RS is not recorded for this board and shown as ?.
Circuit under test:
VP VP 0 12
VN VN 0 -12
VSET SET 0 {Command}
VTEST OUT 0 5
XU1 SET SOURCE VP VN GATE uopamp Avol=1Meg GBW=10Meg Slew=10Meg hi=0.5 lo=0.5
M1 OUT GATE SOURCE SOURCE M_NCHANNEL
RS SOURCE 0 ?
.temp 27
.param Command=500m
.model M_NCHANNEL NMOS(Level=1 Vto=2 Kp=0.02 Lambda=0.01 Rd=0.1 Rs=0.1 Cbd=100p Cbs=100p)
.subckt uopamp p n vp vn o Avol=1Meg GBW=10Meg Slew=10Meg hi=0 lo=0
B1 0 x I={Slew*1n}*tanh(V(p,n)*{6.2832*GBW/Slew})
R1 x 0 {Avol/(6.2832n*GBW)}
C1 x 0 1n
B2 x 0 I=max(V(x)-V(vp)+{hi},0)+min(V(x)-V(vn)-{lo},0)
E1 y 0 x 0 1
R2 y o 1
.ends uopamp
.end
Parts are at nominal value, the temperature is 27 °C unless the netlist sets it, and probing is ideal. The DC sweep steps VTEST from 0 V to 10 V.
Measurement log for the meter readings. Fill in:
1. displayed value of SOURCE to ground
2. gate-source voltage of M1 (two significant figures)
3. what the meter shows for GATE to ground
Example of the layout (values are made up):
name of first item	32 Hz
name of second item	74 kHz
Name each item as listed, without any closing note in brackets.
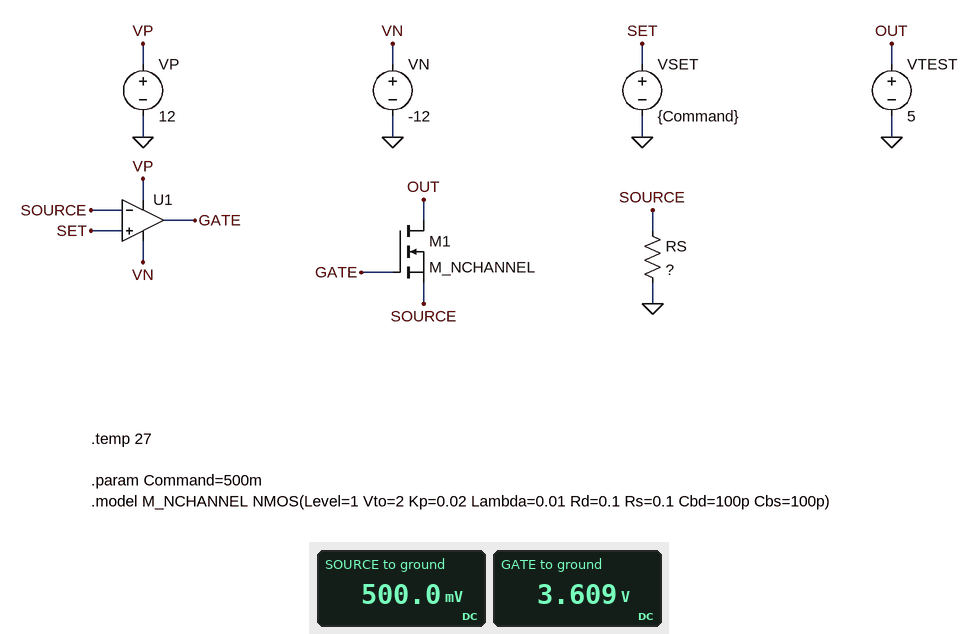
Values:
displayed value of SOURCE to ground	500.0 mV
gate-source voltage of M1	3.1 V
what the meter shows for GATE to ground	3.609 V
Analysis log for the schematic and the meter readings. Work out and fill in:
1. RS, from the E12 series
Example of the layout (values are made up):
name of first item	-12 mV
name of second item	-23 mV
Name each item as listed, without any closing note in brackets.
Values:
RS, from the E12 series	39 Ω
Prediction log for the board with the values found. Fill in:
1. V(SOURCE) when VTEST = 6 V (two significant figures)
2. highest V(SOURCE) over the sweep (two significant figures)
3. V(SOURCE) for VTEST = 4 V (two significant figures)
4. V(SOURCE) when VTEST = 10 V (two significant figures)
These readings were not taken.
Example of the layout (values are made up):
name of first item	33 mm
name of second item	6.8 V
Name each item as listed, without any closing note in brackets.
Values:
V(SOURCE) when VTEST = 6 V	500 mV
highest V(SOURCE) over the sweep	500 mV
V(SOURCE) for VTEST = 4 V	500 mV
V(SOURCE) when VTEST = 10 V	500 mV
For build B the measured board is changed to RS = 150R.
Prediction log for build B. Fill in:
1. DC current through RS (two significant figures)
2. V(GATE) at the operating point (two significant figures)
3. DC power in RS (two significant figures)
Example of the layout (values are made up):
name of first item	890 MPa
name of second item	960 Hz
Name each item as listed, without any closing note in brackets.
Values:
DC current through RS	3.3 mA
V(GATE) at the operating point	3.1 V
DC power in RS	1.7 mW
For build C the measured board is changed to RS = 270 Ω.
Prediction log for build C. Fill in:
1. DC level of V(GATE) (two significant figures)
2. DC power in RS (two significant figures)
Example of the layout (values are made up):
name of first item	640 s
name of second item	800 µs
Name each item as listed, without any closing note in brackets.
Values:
DC level of V(GATE)	2.9 V
DC power in RS	930 µW
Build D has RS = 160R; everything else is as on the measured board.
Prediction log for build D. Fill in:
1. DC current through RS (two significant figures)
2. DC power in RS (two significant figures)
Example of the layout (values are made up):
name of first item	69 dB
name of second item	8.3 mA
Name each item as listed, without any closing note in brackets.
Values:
DC current through RS	3.1 mA
DC power in RS	1.6 mW
